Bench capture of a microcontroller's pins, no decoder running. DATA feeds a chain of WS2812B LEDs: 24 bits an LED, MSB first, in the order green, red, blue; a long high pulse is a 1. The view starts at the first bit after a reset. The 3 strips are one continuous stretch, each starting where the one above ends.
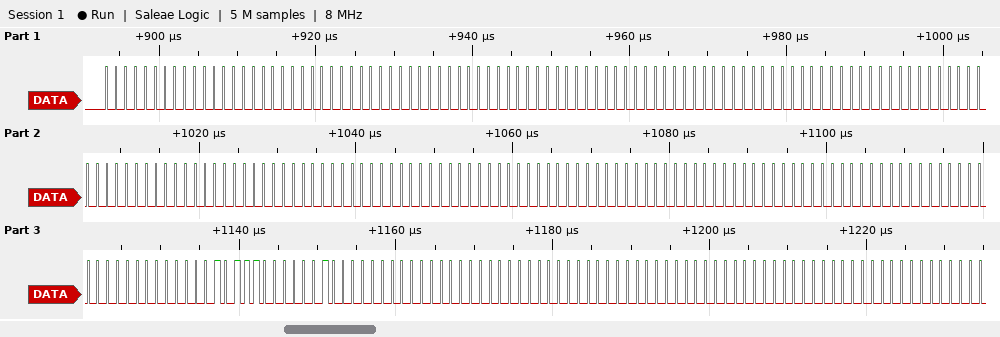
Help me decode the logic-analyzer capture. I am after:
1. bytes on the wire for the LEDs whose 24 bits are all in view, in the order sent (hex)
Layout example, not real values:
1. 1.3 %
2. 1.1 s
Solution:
1. 00 00 00 00 00 00 00 00 00 00 00 00 00 00 00 00 00 00 00 00 00 00 00 00 17 02 00 00 00 00 00 00 00
